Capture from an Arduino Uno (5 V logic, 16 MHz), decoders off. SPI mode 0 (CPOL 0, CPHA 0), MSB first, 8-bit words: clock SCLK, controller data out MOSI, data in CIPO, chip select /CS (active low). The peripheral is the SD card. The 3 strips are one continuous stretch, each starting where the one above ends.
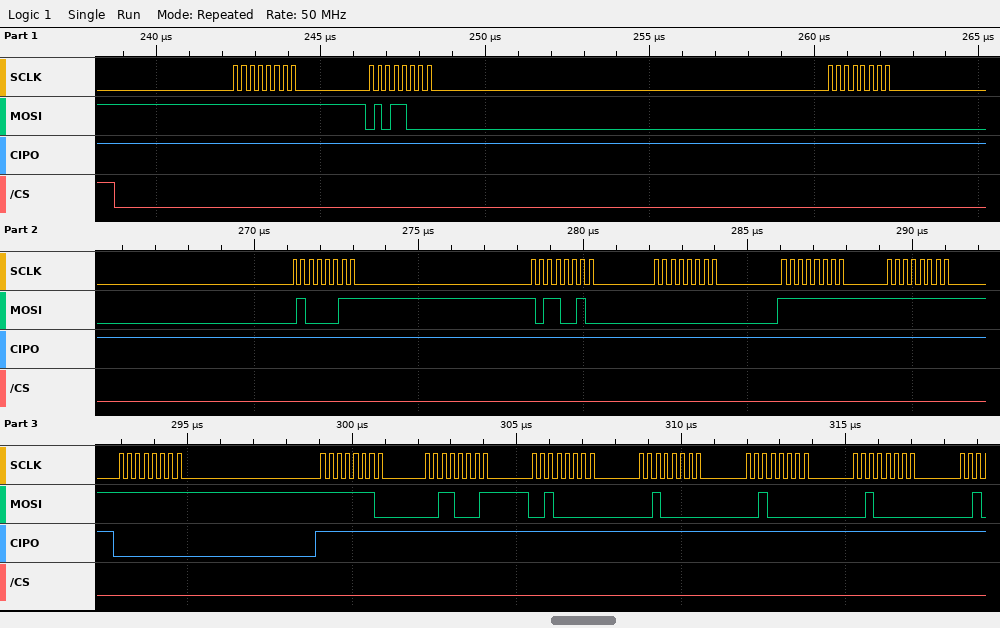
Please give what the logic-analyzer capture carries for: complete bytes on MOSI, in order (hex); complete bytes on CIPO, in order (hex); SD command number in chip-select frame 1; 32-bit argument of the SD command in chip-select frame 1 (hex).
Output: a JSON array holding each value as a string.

["FF 58 00 43 B2 00 FF FF FF FE 31 20 20 20 20", "FF FF FF FF FF FF FF FF 00 FF FF FF FF FF FF", "CMD24", "0x0043B200"]
